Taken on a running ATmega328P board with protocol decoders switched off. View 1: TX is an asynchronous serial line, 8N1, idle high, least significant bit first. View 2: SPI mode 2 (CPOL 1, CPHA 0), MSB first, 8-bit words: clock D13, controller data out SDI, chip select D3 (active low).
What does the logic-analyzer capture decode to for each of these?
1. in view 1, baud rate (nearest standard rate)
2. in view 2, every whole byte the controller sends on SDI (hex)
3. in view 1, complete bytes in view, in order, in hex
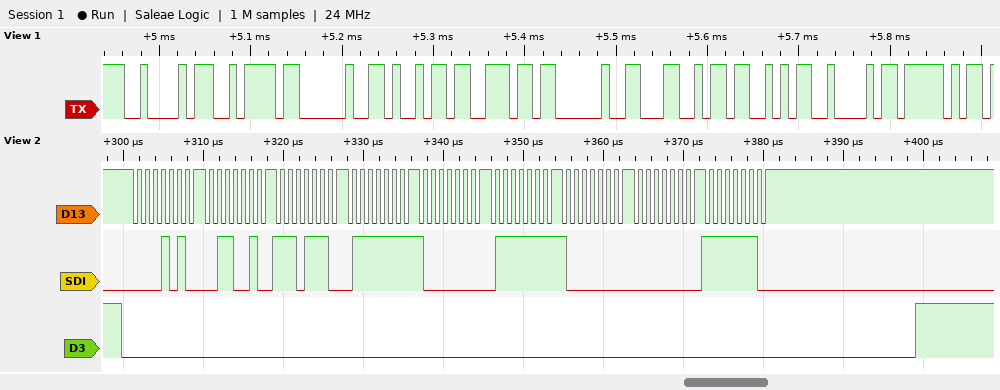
115200 baud
0A 32 EE 7F 80 7F 80 00 FE
42 7A 20 69 6E 20 4C 53 42 5F
